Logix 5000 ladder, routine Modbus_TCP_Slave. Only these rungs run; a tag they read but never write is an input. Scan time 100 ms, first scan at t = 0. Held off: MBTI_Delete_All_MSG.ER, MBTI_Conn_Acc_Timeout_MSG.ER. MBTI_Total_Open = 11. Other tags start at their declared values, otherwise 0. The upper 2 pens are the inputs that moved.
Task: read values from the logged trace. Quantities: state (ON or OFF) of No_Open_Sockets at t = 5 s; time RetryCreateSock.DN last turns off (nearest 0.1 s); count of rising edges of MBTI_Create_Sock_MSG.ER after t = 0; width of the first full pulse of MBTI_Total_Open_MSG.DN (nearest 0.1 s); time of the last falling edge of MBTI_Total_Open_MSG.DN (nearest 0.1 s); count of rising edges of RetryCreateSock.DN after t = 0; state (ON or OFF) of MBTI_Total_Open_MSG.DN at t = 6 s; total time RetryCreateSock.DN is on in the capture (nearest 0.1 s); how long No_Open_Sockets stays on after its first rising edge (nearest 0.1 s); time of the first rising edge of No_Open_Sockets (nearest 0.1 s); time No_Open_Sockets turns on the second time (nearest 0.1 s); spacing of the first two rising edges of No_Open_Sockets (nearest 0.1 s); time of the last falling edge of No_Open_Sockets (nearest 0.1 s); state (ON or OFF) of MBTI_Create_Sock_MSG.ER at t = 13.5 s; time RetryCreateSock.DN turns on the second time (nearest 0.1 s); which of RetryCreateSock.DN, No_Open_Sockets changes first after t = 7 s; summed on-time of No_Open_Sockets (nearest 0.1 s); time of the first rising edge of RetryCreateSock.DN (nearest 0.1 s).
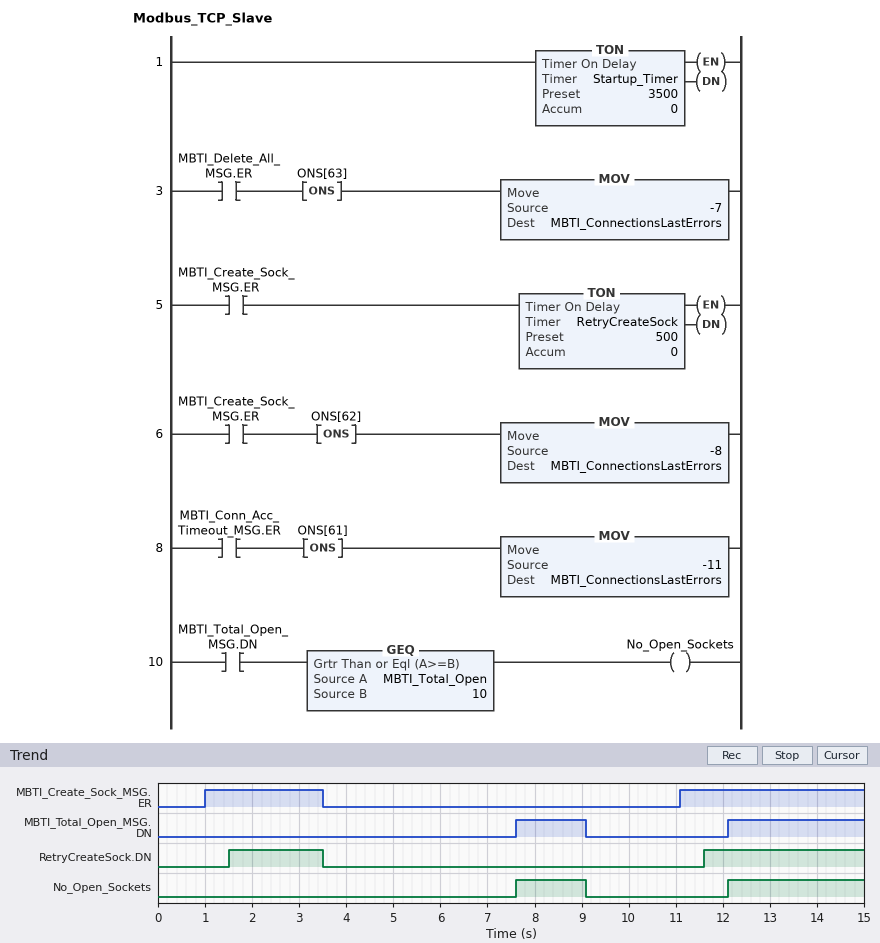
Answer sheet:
OFF
3.5 s
2
1.5 s
9.1 s
2
OFF
5.4 s
1.5 s
7.6 s
12.1 s
4.5 s
9.1 s
ON
11.6 s
No_Open_Sockets
4.4 s
1.5 s
